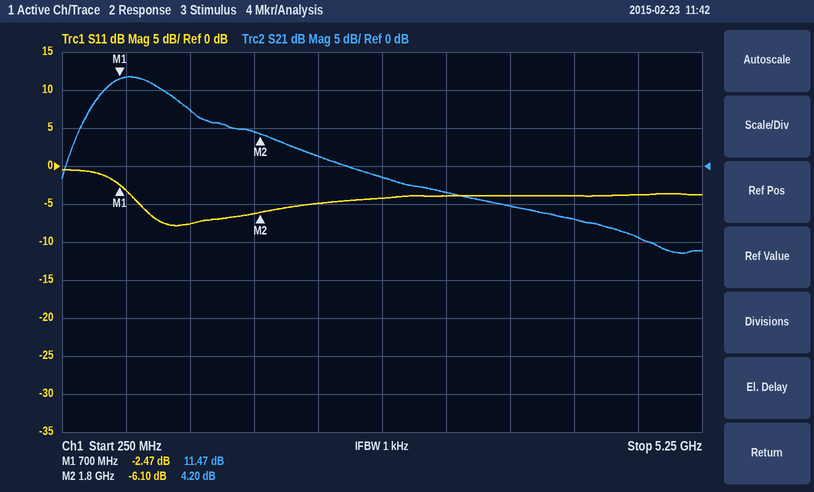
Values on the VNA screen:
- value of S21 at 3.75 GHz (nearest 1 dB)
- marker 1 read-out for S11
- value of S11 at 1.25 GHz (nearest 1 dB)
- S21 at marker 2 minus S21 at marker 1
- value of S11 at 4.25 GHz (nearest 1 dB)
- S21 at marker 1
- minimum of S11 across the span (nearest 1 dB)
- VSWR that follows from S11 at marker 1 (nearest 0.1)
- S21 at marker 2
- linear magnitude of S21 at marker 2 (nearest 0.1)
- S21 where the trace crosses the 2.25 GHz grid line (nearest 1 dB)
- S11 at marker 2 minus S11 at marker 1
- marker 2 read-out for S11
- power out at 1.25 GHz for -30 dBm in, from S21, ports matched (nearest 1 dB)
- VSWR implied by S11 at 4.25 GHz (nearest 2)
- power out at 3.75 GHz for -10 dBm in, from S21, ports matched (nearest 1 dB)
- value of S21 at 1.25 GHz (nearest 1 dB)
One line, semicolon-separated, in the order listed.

-5 dB; -2.47 dB; -8 dB; -7.27 dB; -4 dB; 11.47 dB; -8 dB; 7.1; 4.20 dB; 1.6; 1 dB; -3.63 dB; -6.10 dB; -23 dBm; 4; -15 dBm; 7 dB
